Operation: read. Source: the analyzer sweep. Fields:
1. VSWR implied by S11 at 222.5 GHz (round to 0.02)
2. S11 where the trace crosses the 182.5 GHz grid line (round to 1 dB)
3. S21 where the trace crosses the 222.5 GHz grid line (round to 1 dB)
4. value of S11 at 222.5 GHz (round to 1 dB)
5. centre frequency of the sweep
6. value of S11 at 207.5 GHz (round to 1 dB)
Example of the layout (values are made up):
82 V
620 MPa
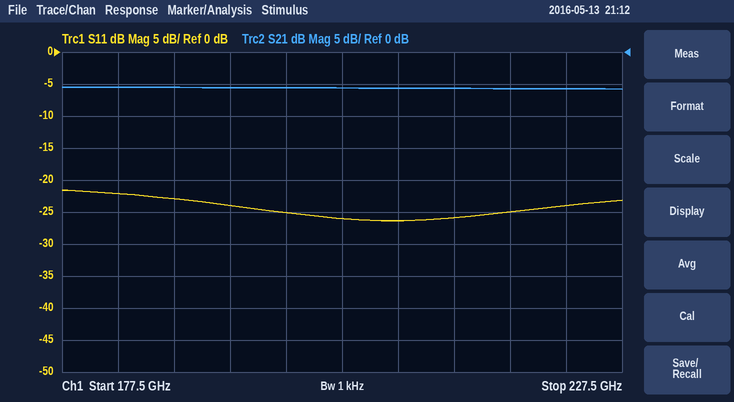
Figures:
1.14
-22 dB
-6 dB
-24 dB
202.5 GHz
-26 dB
